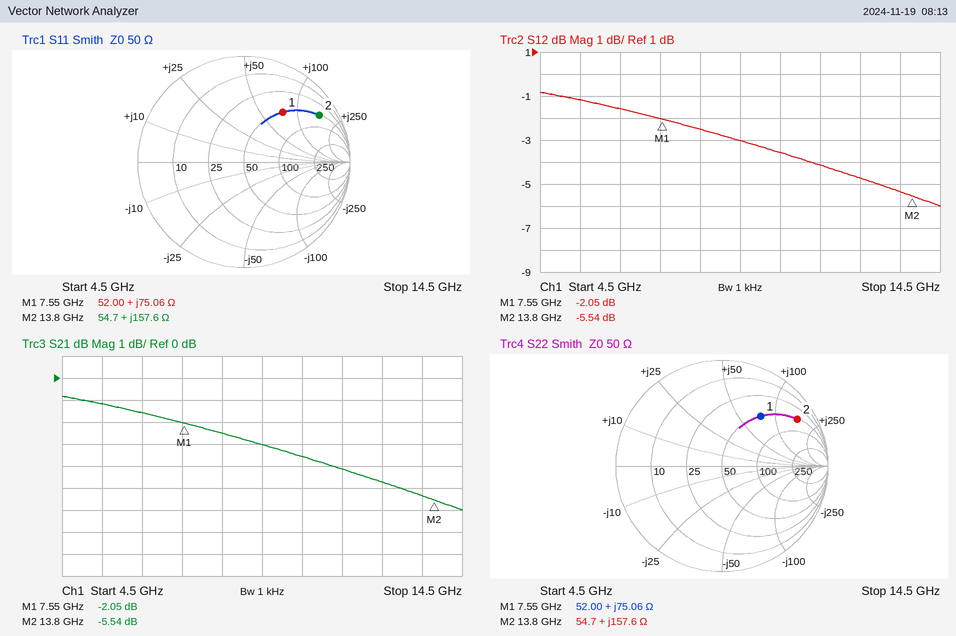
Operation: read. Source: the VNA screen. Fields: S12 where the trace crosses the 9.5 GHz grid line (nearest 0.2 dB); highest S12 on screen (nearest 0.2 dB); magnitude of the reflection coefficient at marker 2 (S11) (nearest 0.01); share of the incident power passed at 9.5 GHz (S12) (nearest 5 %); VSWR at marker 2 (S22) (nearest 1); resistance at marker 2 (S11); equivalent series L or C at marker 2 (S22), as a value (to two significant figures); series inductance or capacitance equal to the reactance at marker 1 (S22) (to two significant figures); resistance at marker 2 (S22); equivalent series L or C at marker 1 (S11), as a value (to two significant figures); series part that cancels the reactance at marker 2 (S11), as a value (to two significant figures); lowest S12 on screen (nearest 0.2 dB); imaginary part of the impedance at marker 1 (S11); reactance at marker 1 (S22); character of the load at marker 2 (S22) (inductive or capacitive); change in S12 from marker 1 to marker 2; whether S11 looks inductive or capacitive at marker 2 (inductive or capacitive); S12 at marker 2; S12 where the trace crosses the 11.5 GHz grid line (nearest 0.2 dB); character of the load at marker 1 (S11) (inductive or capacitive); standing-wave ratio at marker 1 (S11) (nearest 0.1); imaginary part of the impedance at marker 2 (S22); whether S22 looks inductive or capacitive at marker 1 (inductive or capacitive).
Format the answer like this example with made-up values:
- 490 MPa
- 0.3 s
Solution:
- -3.0 dB
- -0.8 dB
- 0.83
- 50 %
- 11
- 54.7 Ω
- 1.8 nH
- 1.6 nH
- 54.7 Ω
- 1.6 nH
- 73 fF
- -6.0 dB
- +75.06 Ω
- +75.06 Ω
- inductive
- -3.49 dB
- inductive
- -5.54 dB
- -4.2 dB
- inductive
- 3.9
- +157.6 Ω
- inductive
